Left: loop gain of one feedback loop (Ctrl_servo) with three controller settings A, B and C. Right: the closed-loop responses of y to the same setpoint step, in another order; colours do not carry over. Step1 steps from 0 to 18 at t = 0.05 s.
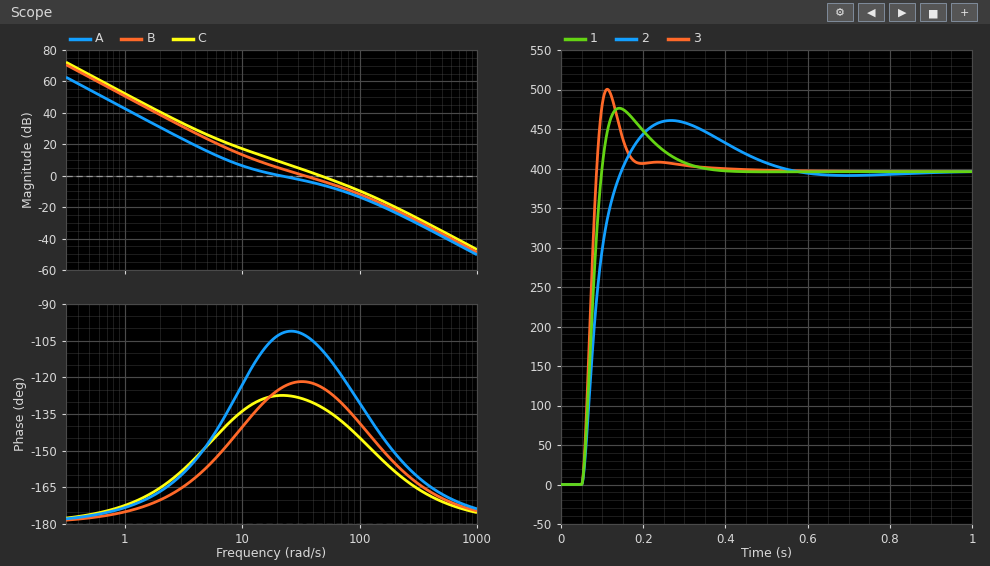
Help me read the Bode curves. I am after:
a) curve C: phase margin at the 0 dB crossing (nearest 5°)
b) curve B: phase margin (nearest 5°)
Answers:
50°
60°
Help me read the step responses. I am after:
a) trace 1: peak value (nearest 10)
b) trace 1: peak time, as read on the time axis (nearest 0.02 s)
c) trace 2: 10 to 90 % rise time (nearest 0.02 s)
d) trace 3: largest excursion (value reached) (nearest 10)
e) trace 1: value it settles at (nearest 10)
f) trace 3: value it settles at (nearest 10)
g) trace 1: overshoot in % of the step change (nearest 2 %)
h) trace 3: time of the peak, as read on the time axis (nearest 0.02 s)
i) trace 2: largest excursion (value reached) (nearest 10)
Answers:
480
0.14 s
0.06 s
500
400
400
20 %
0.12 s
460
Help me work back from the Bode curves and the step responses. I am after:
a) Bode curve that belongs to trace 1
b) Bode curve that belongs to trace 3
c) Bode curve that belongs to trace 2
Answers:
B
C
A
